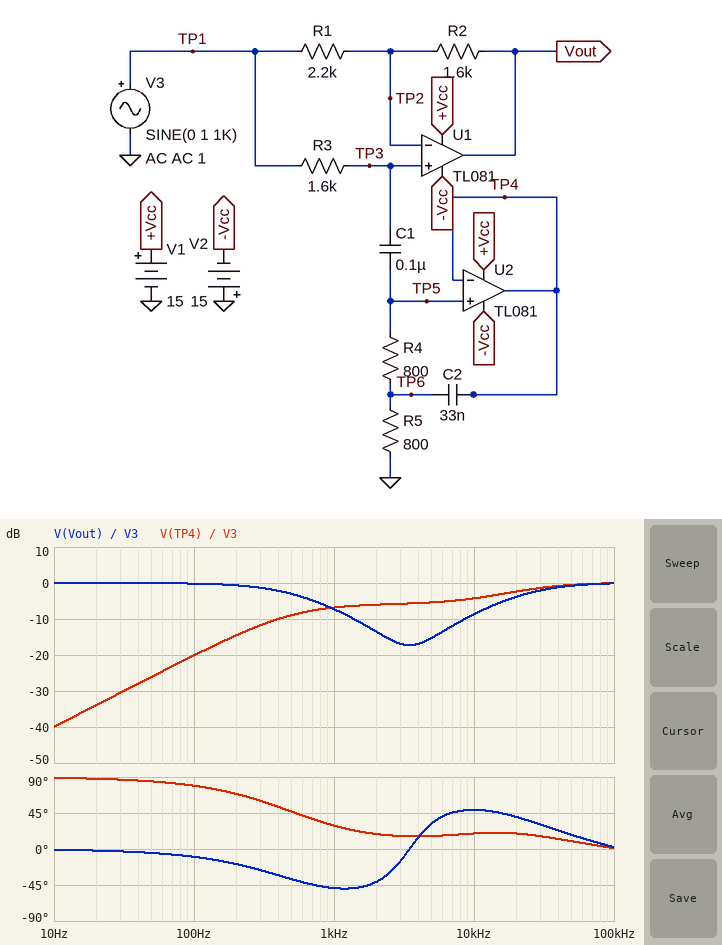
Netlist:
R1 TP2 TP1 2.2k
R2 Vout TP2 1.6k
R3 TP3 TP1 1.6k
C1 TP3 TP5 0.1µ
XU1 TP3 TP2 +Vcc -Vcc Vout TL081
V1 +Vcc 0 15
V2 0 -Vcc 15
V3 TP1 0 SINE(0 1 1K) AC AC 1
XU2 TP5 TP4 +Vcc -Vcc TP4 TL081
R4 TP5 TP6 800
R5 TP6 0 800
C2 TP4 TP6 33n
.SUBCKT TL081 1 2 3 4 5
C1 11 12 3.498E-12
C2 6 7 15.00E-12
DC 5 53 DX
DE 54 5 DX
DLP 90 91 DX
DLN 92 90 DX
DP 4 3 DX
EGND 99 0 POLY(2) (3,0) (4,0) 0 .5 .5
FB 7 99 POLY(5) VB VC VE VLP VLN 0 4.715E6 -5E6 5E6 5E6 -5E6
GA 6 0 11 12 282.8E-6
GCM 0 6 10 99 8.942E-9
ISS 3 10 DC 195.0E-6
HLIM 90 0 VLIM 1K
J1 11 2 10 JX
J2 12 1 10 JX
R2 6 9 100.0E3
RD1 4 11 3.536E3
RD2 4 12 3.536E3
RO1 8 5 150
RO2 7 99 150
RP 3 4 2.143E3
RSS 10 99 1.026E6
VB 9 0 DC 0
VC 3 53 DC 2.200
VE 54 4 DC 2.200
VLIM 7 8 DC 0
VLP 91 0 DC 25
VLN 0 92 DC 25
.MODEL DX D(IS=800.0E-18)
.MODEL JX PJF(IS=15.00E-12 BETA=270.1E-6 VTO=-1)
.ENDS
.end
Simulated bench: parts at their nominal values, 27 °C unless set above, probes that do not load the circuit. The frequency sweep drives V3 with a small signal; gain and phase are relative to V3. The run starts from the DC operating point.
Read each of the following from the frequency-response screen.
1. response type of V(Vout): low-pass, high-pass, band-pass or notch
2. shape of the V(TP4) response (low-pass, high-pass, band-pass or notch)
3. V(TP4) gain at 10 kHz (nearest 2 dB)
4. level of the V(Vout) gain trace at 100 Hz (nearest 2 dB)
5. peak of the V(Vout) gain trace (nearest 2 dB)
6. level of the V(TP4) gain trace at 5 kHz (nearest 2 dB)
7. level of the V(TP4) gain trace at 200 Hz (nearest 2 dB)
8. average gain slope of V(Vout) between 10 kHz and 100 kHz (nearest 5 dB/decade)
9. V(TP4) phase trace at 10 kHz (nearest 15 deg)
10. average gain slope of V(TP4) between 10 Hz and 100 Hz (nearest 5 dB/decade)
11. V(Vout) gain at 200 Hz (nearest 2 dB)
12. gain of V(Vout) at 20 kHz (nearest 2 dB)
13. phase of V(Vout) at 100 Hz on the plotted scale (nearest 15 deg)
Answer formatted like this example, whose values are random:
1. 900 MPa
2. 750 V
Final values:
1. notch
2. high-pass
3. -4 dB
4. 0 dB
5. 0 dB
6. -6 dB
7. -14 dB
8. 10 dB/decade
9. 15 deg
10. 20 dB/decade
11. 0 dB
12. -4 dB
13. -15 deg
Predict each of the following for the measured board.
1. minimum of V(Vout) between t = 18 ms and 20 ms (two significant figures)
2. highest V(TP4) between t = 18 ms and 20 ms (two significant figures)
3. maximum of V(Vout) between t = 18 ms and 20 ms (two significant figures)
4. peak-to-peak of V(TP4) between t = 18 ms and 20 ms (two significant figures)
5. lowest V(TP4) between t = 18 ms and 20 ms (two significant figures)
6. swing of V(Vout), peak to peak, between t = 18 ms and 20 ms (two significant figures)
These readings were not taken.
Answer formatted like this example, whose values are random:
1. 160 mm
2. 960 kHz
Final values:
1. -430 mV
2. 460 mV
3. 430 mV
4. 910 mV
5. -460 mV
6. 870 mV
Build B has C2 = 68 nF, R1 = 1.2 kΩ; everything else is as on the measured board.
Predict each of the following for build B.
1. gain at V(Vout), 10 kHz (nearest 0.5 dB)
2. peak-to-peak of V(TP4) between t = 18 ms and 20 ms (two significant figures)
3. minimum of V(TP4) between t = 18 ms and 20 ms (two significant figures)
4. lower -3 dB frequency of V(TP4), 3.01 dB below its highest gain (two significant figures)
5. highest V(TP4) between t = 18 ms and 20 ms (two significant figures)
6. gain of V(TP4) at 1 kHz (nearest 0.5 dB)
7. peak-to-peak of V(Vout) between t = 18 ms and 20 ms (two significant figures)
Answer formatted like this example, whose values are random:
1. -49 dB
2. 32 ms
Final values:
1. -4.0 dB
2. 940 mV
3. -470 mV
4. 7.5 kHz
5. 470 mV
6. -6.5 dB
7. 820 mV
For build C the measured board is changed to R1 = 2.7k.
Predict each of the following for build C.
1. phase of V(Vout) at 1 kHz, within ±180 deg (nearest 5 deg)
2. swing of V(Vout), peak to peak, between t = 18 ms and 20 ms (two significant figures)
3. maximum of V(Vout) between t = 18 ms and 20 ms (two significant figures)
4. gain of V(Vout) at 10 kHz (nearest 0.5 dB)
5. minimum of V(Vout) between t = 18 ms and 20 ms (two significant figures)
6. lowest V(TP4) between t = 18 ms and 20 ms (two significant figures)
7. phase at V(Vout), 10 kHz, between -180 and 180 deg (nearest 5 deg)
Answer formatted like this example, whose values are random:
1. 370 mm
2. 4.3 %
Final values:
1. -40 deg
2. 910 mV
3. 450 mV
4. -8.0 dB
5. -450 mV
6. -460 mV
7. 40 deg
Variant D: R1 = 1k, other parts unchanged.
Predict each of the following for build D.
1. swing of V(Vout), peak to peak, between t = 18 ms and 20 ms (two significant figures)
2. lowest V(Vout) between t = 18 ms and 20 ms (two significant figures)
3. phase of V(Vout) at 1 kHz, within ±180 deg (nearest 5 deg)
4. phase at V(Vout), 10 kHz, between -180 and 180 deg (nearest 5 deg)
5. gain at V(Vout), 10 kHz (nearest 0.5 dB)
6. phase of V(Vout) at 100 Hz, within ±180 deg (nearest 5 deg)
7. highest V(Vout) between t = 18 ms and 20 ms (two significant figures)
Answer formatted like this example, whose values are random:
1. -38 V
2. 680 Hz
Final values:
1. 990 mV
2. -500 mV
3. -100 deg
4. 110 deg
5. -7.0 dB
6. -15 deg
7. 500 mV
